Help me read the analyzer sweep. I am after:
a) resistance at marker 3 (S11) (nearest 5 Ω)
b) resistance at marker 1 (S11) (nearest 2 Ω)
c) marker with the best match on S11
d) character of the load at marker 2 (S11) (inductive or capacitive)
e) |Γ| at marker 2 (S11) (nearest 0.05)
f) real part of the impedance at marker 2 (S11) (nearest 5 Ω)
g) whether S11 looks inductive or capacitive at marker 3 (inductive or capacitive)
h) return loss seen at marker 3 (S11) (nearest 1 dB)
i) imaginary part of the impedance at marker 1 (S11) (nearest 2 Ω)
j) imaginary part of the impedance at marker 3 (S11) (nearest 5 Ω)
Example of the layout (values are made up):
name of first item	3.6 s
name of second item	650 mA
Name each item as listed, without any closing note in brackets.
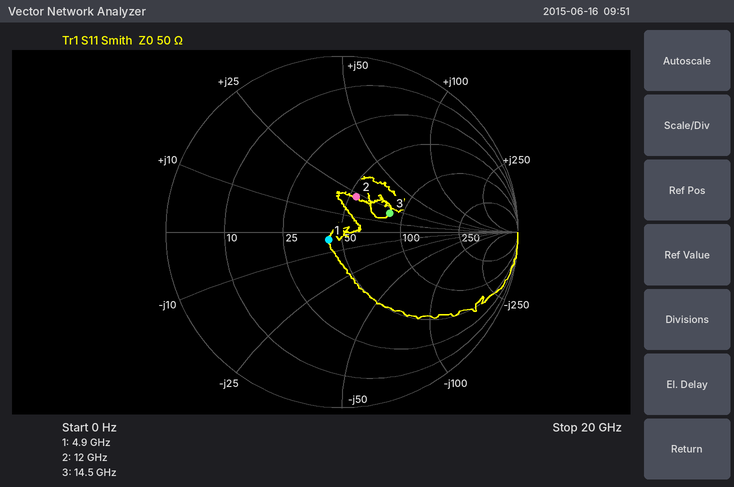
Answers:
resistance at marker 3 (S11)	85 Ω
resistance at marker 1 (S11)	42 Ω
marker with the best match on S11	marker 1
character of the load at marker 2 (S11)	inductive
|Γ| at marker 2 (S11)	0.20
real part of the impedance at marker 2 (S11)	55 Ω
whether S11 looks inductive or capacitive at marker 3	inductive
return loss seen at marker 3 (S11)	11 dB
imaginary part of the impedance at marker 1 (S11)	-4 Ω
imaginary part of the impedance at marker 3 (S11)	+20 Ω
